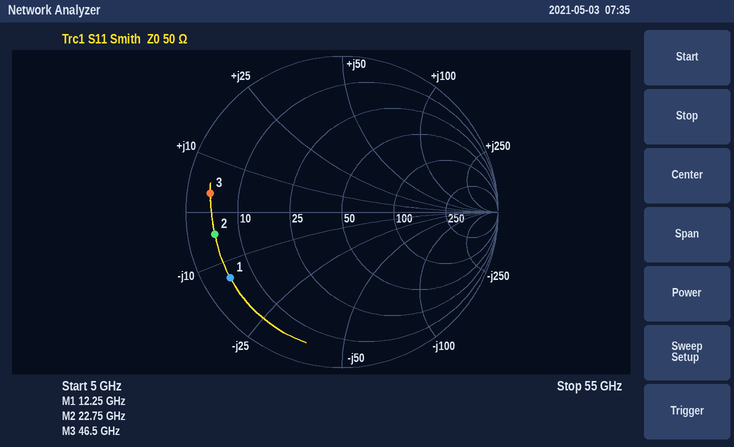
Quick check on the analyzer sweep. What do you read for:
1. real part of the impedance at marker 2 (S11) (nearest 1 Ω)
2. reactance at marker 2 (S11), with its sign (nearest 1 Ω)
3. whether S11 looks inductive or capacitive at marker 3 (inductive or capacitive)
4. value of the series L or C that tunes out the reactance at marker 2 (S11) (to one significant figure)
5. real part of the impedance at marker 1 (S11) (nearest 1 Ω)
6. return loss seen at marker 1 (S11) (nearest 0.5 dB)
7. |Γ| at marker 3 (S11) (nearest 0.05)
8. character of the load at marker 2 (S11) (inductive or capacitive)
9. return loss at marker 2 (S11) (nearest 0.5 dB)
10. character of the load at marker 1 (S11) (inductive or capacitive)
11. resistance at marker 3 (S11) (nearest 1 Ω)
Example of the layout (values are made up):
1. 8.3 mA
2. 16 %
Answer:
1. 5 Ω
2. -4 Ω
3. inductive
4. 30 pH
5. 5 Ω
6. 1.5 dB
7. 0.85
8. capacitive
9. 1.5 dB
10. capacitive
11. 4 Ω
